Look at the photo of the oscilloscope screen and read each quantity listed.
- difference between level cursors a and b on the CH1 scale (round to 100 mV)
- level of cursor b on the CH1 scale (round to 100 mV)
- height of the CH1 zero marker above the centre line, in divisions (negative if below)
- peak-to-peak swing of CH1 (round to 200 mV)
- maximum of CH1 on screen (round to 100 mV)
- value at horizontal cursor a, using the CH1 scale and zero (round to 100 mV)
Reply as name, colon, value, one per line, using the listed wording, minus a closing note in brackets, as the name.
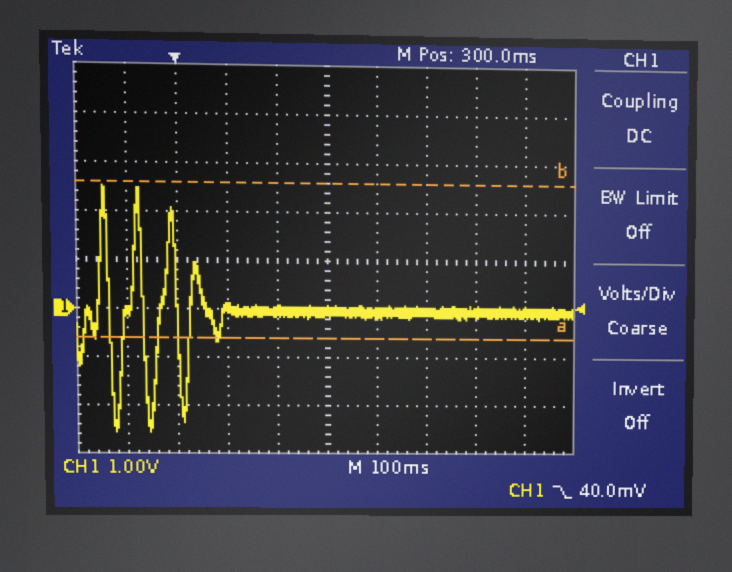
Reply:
difference between level cursors a and b on the CH1 scale: 3.2 V
level of cursor b on the CH1 scale: 2.6 V
height of the CH1 zero marker above the centre line, in divisions: -1.0 div
peak-to-peak swing of CH1: 5.0 V
maximum of CH1 on screen: 2.5 V
value at horizontal cursor a, using the CH1 scale and zero: -600 mV
